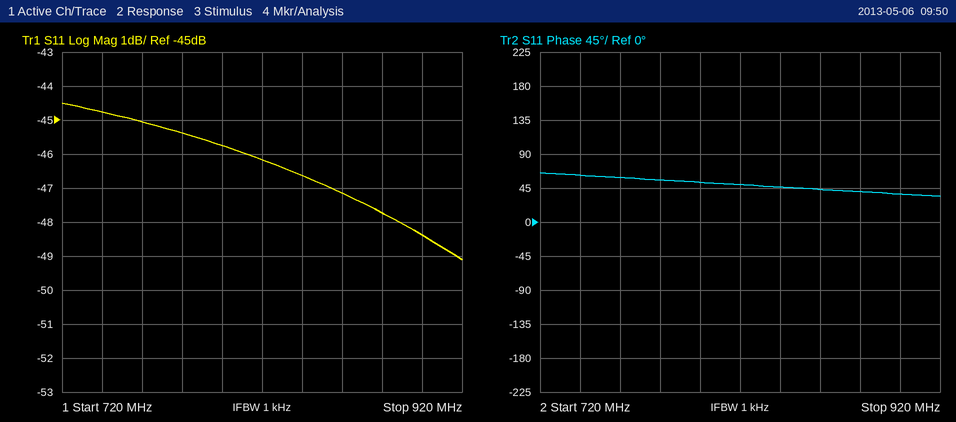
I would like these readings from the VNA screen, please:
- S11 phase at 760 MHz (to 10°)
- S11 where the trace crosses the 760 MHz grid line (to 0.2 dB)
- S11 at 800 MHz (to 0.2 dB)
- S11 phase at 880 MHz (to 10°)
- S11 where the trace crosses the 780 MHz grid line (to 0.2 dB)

60°
-45.0 dB
-45.8 dB
40°
-45.4 dB
